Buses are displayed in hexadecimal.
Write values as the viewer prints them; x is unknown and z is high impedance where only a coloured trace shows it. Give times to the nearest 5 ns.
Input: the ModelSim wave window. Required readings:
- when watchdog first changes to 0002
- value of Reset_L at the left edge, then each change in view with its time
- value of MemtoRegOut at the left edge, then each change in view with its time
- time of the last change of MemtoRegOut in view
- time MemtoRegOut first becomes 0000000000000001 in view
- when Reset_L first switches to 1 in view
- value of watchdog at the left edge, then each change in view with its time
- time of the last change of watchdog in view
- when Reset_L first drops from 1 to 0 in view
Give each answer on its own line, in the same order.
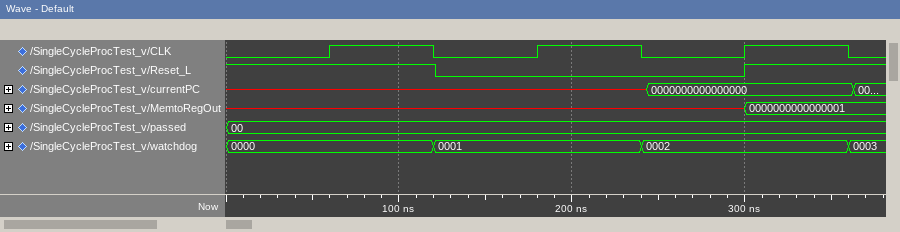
240 ns
1, 0 at 120 ns, 1 at 300 ns
x, 0000000000000001 at 300 ns
300 ns
300 ns
300 ns
0000, 0001 at 120 ns, 0002 at 240 ns, 0003 at 360 ns
360 ns
120 ns
